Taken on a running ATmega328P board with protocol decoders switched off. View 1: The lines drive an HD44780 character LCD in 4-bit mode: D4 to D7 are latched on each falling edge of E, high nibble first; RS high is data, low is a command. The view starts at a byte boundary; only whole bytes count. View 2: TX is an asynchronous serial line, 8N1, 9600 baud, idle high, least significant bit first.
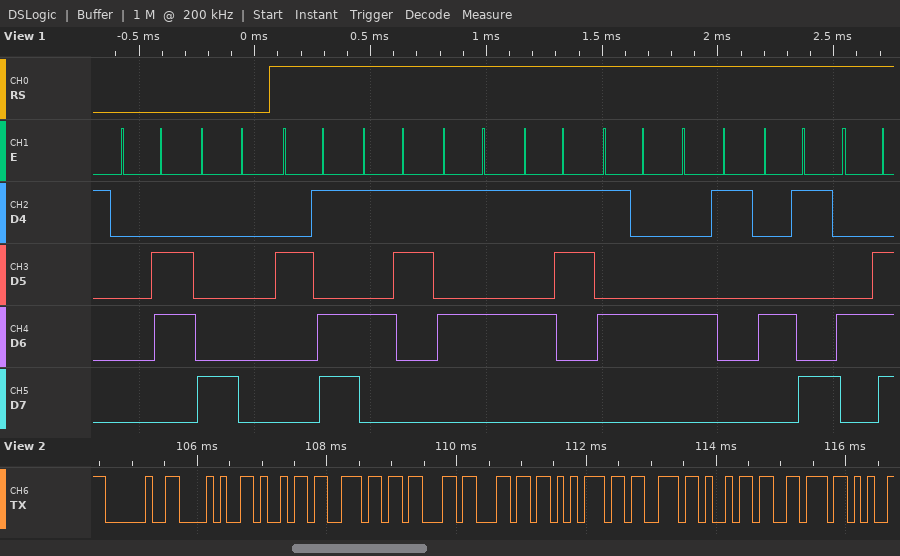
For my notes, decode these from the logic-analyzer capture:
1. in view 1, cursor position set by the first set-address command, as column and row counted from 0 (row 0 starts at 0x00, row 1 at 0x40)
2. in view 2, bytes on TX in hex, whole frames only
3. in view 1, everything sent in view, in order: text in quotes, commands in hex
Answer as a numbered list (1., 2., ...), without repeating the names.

1. column 0, row 0
2. 20 28 69 6E 63 6C 75 73 69 76
3. 0x06 0x80 "-SUSTAIN"
